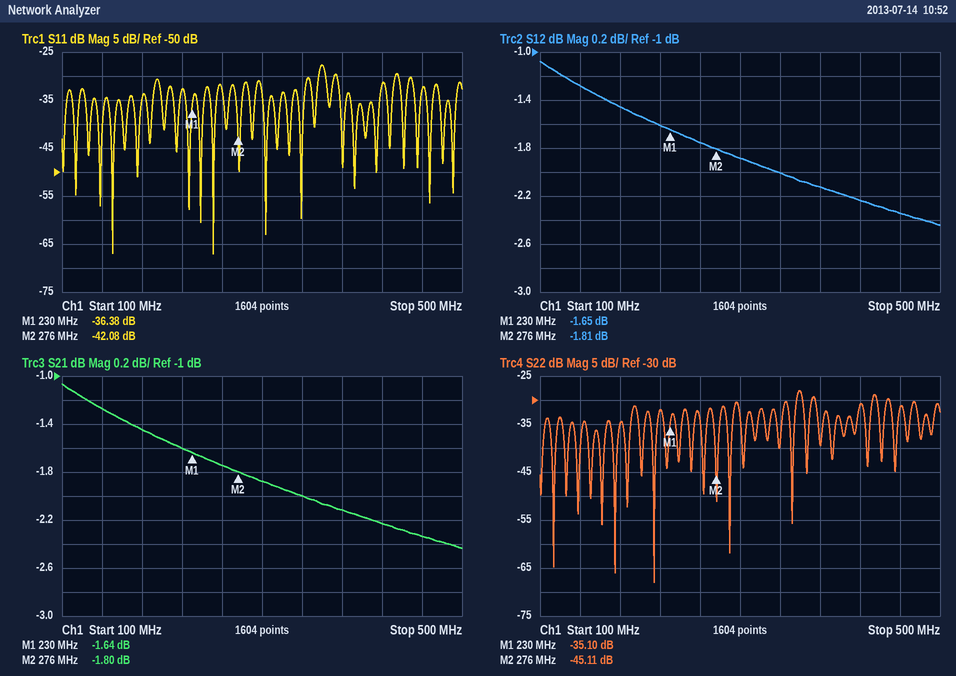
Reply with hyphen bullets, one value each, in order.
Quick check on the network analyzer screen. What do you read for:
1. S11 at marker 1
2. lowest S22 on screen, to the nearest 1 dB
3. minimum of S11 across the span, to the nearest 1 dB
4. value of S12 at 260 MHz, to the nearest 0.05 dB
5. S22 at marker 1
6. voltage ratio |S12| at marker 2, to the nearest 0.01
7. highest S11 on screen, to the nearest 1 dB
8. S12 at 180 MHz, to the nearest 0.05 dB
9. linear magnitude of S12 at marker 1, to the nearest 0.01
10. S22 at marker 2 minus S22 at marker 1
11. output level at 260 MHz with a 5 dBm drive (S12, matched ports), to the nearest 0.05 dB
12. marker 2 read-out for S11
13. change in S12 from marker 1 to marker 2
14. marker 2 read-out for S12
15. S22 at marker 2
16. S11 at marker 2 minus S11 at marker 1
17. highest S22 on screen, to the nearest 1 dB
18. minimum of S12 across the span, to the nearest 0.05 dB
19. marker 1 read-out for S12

- -36.38 dB
- -68 dB
- -67 dB
- -1.75 dB
- -35.10 dB
- 0.81
- -28 dB
- -1.45 dB
- 0.83
- -10.01 dB
- 3.25 dBm
- -42.08 dB
- -0.16 dB
- -1.81 dB
- -45.11 dB
- -5.70 dB
- -28 dB
- -2.45 dB
- -1.65 dB
